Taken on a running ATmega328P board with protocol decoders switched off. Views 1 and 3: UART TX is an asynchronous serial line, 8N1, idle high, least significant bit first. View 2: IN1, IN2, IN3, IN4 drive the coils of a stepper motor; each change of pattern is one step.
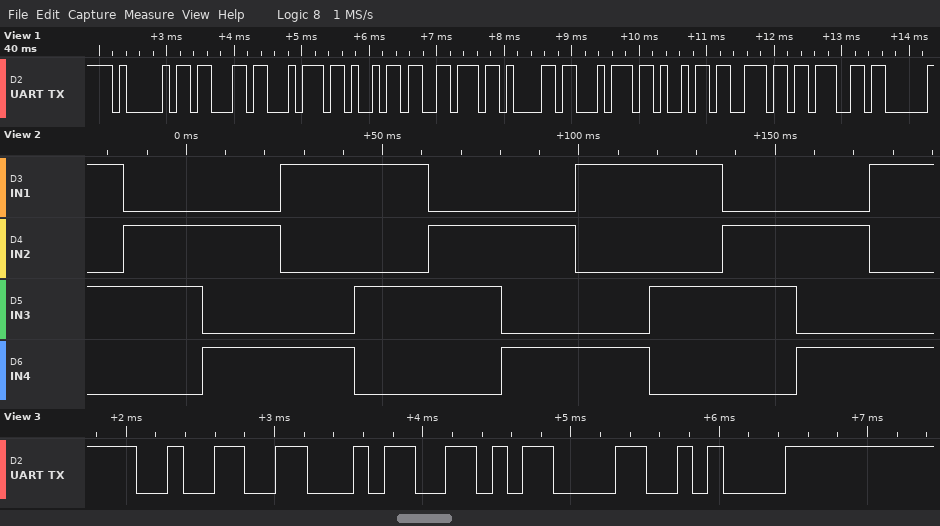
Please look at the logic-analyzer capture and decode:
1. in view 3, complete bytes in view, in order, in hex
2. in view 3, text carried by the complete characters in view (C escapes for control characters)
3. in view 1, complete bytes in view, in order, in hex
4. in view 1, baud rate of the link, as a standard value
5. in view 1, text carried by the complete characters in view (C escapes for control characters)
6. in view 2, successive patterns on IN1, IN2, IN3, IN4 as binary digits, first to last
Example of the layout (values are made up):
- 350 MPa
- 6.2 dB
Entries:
- 0x32 0x34 0x0D 0x0A
- "24\r\n"
- 41 63 74 69 76 61 74 69 6E 67
- 9600 baud
- "Activating"
- 1010 0110 0101 1001 1010 0110 0101 1001 1010 0110 0101 1001
